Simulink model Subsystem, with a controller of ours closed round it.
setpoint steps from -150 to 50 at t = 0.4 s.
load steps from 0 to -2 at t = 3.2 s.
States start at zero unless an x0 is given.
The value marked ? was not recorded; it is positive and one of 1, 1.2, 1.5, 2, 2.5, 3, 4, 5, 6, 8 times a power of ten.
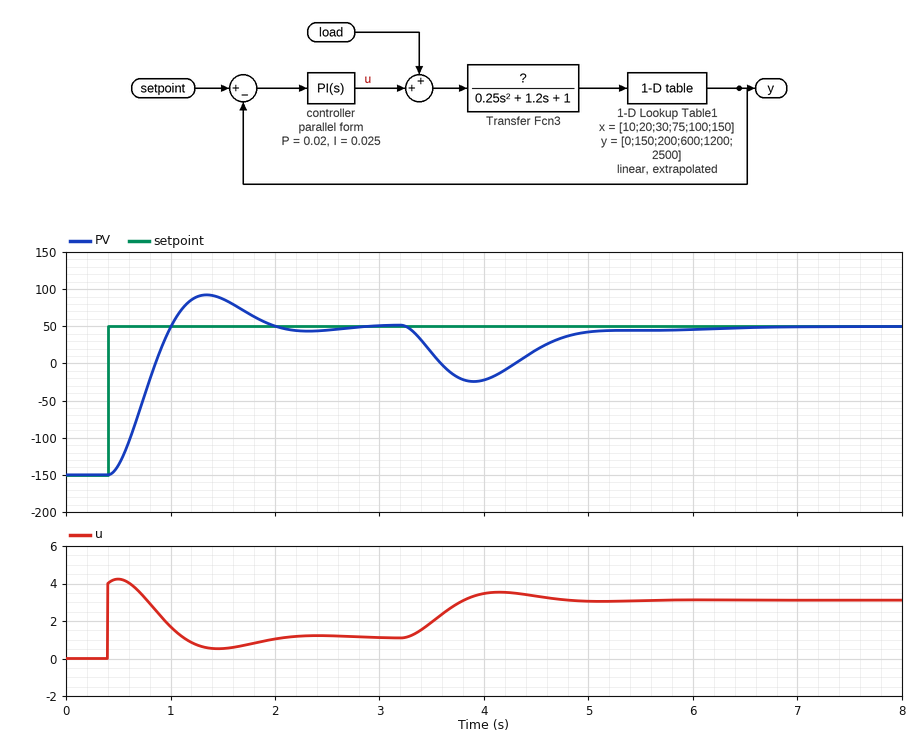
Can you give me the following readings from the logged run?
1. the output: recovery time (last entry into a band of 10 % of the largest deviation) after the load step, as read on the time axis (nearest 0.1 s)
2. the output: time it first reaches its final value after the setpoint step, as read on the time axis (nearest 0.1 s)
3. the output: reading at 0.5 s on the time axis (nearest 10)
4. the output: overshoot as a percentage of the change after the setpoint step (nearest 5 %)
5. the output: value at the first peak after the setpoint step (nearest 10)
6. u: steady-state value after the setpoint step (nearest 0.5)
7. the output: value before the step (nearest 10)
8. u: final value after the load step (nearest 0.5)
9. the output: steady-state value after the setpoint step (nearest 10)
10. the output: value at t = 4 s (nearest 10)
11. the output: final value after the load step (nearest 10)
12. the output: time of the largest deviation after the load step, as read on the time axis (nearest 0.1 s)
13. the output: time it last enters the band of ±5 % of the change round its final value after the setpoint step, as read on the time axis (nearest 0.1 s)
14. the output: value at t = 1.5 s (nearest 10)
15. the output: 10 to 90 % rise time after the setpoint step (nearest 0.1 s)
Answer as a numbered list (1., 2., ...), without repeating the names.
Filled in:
1. 5.0 s
2. 1.0 s
3. -140
4. 20 %
5. 90
6. 1.0
7. -150
8. 3.0
9. 50
10. -20
11. 50
12. 3.9 s
13. 1.8 s
14. 90
15. 0.4 s
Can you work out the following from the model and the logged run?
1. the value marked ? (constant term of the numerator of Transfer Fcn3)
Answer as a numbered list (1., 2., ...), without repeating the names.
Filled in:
1. 12
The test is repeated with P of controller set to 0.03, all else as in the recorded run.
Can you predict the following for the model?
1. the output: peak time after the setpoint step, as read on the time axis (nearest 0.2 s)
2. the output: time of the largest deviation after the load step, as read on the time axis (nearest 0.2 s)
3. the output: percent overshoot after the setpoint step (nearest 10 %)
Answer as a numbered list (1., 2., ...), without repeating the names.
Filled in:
1. 1.2 s
2. 3.8 s
3. 20 %
